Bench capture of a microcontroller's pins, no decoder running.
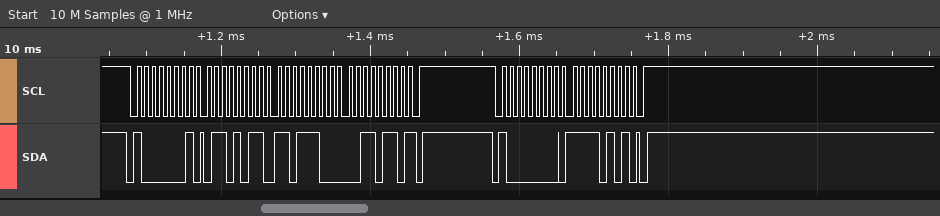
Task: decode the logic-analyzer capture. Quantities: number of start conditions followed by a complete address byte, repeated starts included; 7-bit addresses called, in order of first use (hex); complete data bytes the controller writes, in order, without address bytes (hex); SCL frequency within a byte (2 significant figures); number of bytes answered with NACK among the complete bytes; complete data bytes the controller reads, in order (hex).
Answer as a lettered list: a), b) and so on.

a) 2
b) 0x40
c) F5
d) 100 kHz
e) 1
f) 6B DC 36
